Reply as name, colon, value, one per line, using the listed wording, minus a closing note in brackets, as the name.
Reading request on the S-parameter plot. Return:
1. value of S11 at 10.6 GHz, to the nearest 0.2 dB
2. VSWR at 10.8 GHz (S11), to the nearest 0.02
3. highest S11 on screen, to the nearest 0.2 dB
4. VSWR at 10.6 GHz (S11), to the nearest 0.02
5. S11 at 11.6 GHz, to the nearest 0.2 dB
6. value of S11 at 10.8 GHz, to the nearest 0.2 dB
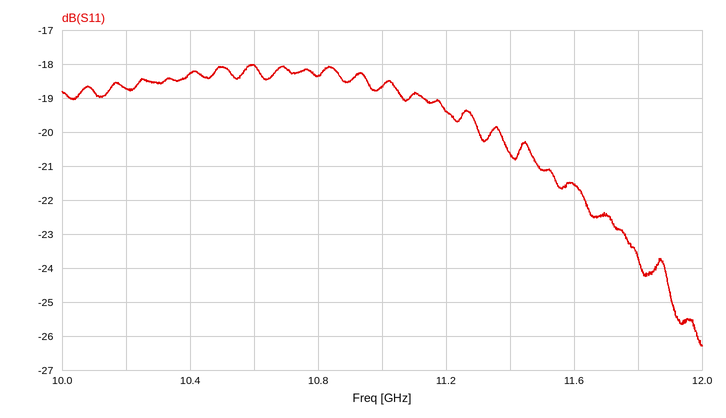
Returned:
value of S11 at 10.6 GHz, to the nearest 0.2 dB: -18.0 dB
VSWR at 10.8 GHz (S11), to the nearest 0.02: 1.28
highest S11 on screen, to the nearest 0.2 dB: -18.0 dB
VSWR at 10.6 GHz (S11), to the nearest 0.02: 1.28
S11 at 11.6 GHz, to the nearest 0.2 dB: -21.6 dB
value of S11 at 10.8 GHz, to the nearest 0.2 dB: -18.4 dB
